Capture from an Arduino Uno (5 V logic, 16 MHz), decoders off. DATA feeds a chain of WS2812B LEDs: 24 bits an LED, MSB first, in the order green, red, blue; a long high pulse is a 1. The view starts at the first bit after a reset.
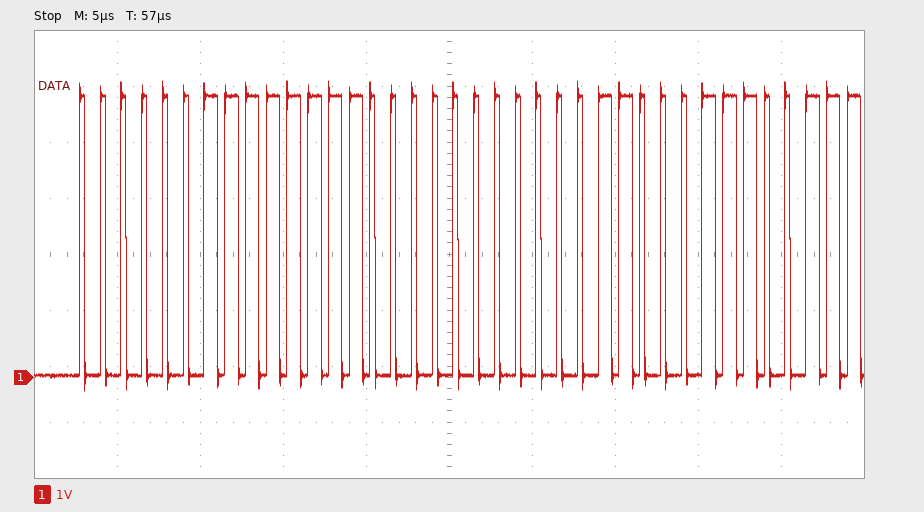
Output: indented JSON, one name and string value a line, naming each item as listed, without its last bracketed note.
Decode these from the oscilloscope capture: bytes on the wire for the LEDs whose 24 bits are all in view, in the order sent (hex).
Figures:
{
  "bytes on the wire for the LEDs whose 24 bits are all in view, in the order sent": "03 FC 00"
}
